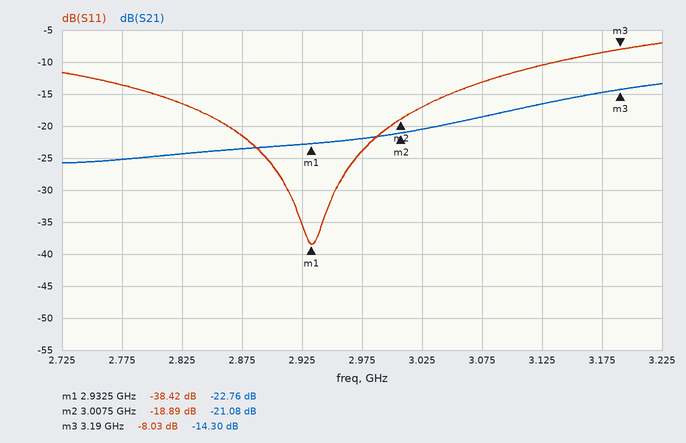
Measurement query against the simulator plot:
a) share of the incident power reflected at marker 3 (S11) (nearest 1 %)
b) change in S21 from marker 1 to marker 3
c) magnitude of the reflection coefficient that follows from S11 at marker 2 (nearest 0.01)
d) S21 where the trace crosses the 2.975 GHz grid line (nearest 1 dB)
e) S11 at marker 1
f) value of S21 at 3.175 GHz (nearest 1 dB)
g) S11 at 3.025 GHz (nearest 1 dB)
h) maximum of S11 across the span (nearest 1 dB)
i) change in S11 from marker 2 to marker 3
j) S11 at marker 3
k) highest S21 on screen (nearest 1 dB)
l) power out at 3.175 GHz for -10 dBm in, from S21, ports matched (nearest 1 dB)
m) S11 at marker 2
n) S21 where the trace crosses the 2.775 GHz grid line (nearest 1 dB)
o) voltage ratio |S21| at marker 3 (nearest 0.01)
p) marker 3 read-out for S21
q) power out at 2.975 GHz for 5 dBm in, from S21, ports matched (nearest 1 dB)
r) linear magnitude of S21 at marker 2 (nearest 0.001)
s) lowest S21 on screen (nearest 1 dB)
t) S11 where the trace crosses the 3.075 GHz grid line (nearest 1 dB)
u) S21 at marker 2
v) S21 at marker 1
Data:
16 %
8.46 dB
0.11
-22 dB
-38.42 dB
-15 dB
-17 dB
-7 dB
10.86 dB
-8.03 dB
-13 dB
-25 dBm
-18.89 dB
-25 dB
0.19
-14.30 dB
-17 dBm
0.088
-26 dB
-13 dB
-21.08 dB
-22.76 dB
